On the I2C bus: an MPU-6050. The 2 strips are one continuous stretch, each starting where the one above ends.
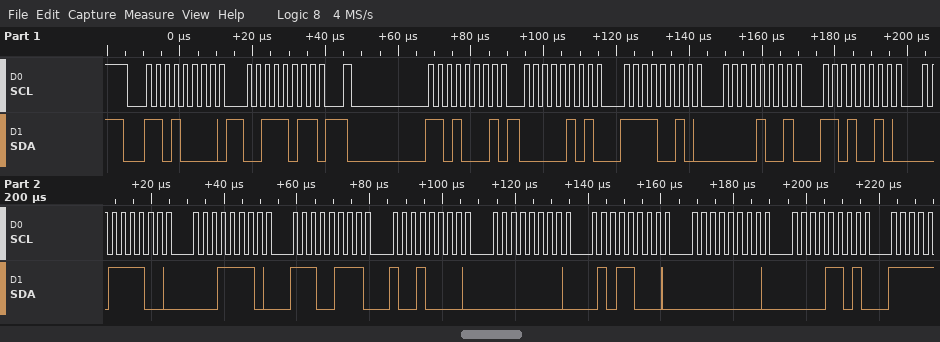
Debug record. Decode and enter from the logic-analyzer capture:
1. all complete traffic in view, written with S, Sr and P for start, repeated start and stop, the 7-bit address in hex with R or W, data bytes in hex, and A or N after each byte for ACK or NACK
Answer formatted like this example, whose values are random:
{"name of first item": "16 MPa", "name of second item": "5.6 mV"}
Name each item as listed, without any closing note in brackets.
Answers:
{"all complete traffic in view, written with S, Sr and P for start, repeated start and stop, the 7-bit address in hex with R or W, data bytes in hex, and A or N after each byte for ACK or NACK": "S 68W A 3B A Sr 68R A 05 A F2 A 09 A D2 A 3C A 1E A E7 A 90 A 00 A 58 A 00 A 0D A"}
